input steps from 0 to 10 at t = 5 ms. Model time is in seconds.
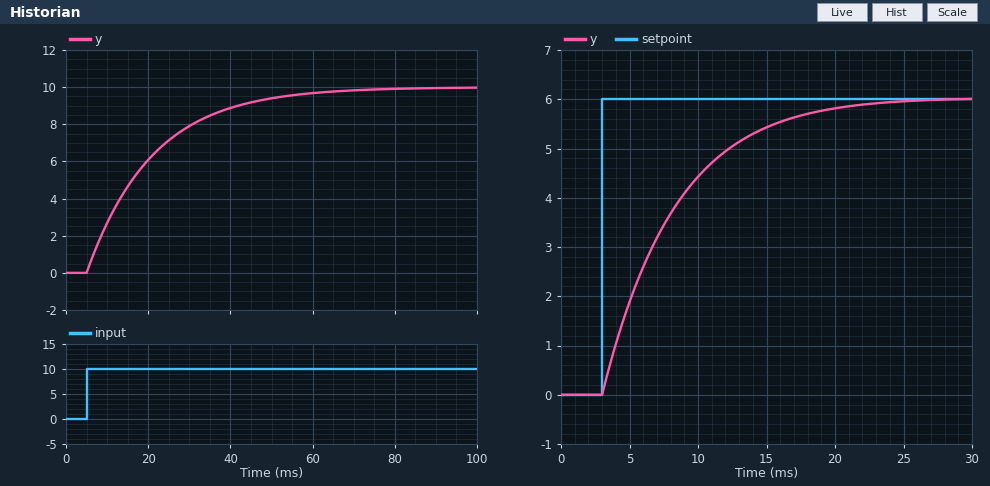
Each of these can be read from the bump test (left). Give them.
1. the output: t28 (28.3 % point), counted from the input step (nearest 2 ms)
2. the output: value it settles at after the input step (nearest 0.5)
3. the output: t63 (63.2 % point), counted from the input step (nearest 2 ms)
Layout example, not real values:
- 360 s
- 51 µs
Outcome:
- 6 ms
- 10.0
- 16 ms
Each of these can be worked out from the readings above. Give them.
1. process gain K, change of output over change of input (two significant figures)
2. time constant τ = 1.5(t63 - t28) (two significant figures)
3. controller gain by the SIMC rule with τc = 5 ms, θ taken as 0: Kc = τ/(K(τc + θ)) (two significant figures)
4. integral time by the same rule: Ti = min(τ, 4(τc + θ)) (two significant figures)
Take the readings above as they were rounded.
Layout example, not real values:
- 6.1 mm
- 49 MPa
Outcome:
- 1.0
- 15 ms
- 3.0
- 15 ms
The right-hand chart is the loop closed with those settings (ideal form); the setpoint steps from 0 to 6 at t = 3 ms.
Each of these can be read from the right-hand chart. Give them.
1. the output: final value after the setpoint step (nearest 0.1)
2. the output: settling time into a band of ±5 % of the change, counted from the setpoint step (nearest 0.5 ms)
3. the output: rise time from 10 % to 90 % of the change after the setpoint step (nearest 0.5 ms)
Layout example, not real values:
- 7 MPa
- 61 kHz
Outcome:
- 6.0
- 15.0 ms
- 11.0 ms
